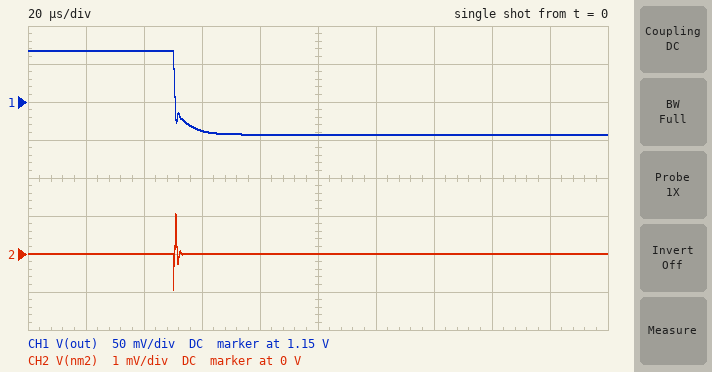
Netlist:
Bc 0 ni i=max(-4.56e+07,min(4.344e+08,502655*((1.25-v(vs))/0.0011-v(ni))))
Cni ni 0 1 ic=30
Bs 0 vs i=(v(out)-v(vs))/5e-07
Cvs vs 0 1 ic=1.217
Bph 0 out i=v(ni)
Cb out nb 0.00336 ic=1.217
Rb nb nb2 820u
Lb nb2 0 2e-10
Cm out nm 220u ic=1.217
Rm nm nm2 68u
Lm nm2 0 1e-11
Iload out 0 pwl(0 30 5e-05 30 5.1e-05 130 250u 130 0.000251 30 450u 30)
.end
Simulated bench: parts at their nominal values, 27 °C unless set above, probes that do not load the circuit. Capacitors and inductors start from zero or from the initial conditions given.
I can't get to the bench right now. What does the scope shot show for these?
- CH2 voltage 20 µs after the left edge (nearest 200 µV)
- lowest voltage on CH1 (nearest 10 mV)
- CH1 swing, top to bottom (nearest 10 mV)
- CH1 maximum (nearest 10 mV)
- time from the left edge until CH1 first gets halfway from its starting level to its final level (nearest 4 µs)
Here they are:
0 V
1.11 V
110 mV
1.22 V
52 µs
